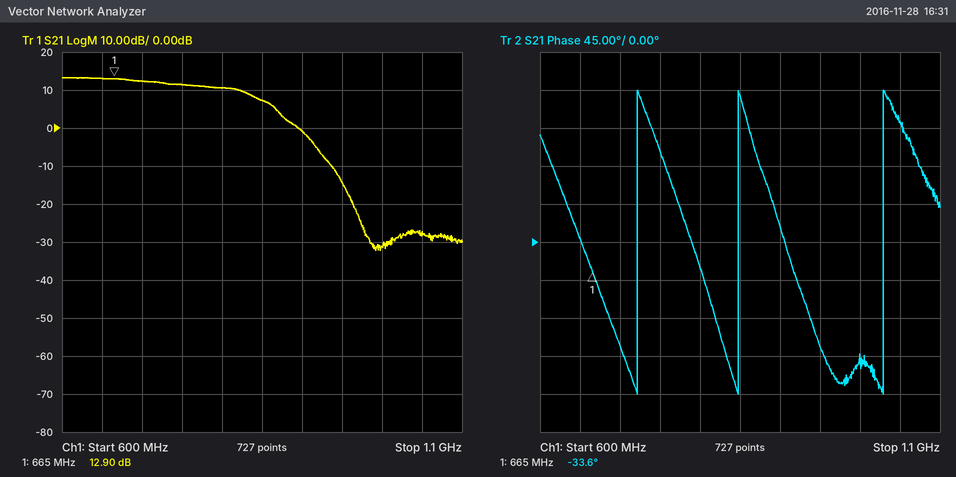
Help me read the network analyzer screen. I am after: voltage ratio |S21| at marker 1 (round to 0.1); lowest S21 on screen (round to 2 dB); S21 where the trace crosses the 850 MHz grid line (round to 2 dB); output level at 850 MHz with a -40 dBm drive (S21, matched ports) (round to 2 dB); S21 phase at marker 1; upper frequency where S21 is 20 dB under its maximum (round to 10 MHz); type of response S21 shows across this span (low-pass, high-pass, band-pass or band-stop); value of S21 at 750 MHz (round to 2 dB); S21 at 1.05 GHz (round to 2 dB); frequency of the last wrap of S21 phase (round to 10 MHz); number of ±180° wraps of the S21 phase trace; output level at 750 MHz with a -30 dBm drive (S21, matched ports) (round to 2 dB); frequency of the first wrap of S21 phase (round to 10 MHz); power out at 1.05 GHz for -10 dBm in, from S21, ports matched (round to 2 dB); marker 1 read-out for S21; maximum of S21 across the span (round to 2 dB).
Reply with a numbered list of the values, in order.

1. 4.4
2. -32 dB
3. 8 dB
4. -32 dBm
5. -33.6°
6. 920 MHz
7. low-pass
8. 12 dB
9. -28 dB
10. 1.03 GHz
11. 3
12. -18 dBm
13. 720 MHz
14. -38 dBm
15. 12.90 dB
16. 14 dB
